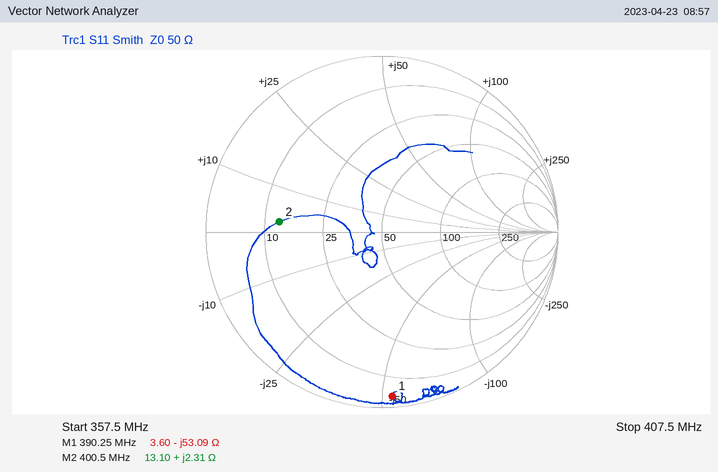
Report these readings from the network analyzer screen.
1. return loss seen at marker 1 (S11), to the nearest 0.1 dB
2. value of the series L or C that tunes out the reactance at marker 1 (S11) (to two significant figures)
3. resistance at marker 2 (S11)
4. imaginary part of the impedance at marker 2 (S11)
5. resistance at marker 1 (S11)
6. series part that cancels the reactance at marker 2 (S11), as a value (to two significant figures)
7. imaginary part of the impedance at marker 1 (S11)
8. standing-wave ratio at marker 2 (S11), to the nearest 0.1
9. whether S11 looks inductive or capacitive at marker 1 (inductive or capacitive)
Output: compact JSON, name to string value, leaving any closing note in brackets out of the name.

{"return loss seen at marker 1 (S11), to the nearest 0.1 dB": "0.6 dB", "value of the series L or C that tunes out the reactance at marker 1 (S11)": "22 nH", "resistance at marker 2": "13.10 Ω", "imaginary part of the impedance at marker 2": "+2.31 Ω", "resistance at marker 1": "3.60 Ω", "series part that cancels the reactance at marker 2 (S11), as a value": "170 pF", "imaginary part of the impedance at marker 1": "-53.09 Ω", "standing-wave ratio at marker 2 (S11), to the nearest 0.1": "3.8", "whether S11 looks inductive or capacitive at marker 1": "capacitive"}
